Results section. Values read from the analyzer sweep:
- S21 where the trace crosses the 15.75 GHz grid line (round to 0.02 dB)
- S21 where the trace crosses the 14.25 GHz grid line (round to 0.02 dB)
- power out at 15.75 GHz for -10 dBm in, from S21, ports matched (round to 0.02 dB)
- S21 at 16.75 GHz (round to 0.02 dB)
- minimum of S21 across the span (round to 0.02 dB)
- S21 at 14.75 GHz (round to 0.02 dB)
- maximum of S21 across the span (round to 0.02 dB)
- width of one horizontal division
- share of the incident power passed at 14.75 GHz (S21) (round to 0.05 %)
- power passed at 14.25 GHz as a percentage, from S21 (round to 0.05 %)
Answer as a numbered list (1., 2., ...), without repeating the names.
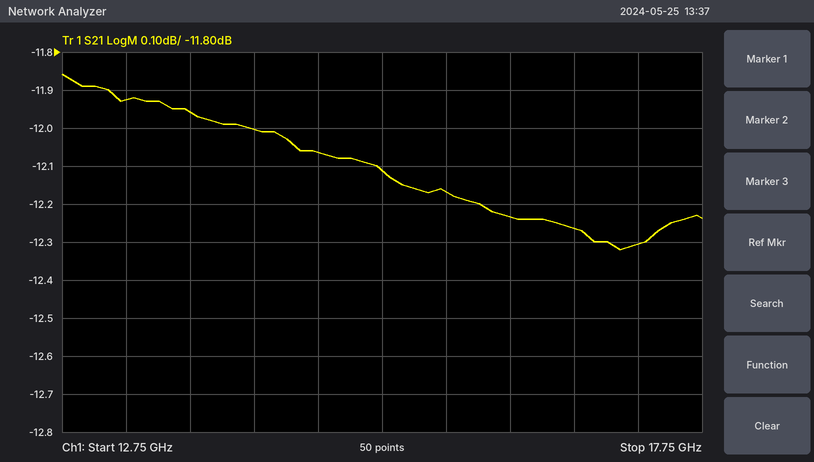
1. -12.16 dB
2. -12.00 dB
3. -22.16 dBm
4. -12.26 dB
5. -12.32 dB
6. -12.06 dB
7. -11.86 dB
8. 500 MHz
9. 6.20 %
10. 6.30 %
